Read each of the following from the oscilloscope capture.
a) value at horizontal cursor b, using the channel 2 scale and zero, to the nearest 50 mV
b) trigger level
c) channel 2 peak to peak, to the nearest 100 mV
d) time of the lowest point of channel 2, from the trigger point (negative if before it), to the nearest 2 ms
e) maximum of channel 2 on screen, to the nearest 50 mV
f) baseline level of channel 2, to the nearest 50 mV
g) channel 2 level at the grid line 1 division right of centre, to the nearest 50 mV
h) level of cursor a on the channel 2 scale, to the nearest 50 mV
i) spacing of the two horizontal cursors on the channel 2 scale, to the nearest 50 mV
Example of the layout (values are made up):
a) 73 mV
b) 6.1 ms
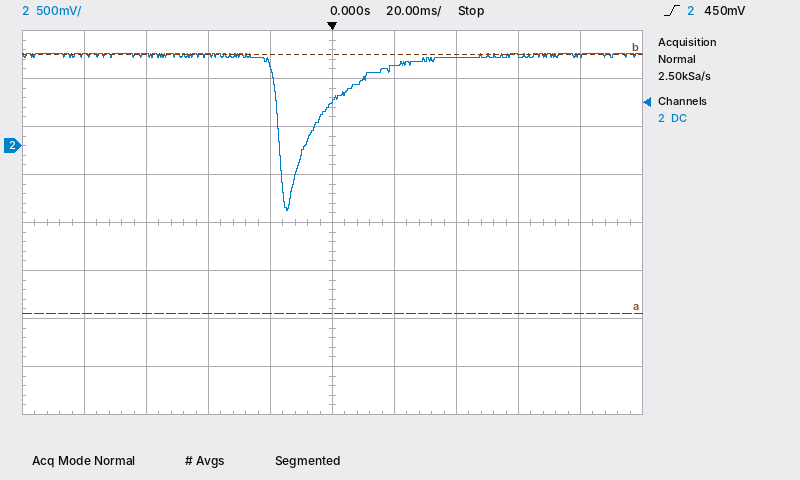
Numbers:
a) 950 mV
b) 450 mV
c) 1.60 V
d) -14 ms
e) 950 mV
f) 950 mV
g) 850 mV
h) -1.75 V
i) 2.70 V
